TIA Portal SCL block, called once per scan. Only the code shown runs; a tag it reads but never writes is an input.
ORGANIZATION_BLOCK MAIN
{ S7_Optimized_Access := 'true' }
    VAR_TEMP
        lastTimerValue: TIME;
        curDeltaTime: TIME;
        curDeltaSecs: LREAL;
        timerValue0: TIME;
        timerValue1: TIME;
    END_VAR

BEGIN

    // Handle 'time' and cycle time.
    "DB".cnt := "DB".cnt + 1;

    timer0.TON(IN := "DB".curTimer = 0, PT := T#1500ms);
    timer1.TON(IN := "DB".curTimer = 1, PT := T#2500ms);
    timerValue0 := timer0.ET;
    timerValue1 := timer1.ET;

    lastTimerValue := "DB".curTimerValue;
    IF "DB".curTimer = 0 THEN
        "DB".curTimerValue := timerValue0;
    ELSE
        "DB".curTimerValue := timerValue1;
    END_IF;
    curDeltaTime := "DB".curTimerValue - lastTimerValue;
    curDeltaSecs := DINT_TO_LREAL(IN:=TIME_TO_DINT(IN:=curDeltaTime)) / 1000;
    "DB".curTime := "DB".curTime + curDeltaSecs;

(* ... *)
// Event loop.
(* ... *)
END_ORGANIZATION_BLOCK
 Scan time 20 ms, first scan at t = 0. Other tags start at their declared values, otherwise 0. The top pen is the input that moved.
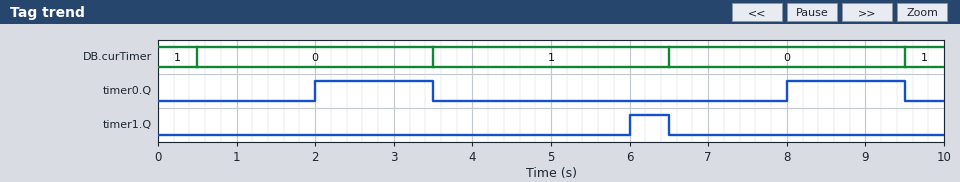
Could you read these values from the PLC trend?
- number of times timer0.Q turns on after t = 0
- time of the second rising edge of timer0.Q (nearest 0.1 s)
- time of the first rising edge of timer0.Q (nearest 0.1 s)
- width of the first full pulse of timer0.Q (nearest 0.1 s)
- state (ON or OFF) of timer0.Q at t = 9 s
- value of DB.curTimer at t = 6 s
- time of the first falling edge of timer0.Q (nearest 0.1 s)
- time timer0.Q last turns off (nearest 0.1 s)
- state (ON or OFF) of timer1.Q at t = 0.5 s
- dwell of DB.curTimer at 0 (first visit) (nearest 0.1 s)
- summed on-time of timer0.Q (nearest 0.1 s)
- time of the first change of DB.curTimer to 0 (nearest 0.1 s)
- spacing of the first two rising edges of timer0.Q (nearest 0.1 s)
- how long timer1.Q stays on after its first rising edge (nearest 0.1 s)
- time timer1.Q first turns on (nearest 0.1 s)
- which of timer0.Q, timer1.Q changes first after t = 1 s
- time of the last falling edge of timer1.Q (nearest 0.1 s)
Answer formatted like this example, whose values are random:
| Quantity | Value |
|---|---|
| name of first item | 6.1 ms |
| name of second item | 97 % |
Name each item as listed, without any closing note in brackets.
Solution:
| Quantity | Value |
|---|---|
| number of times timer0.Q turns on after t = 0 | 2 |
| time of the second rising edge of timer0.Q | 8.0 s |
| time of the first rising edge of timer0.Q | 2.0 s |
| width of the first full pulse of timer0.Q | 1.5 s |
| state (ON or OFF) of timer0.Q at t = 9 s | ON |
| value of DB.curTimer at t = 6 s | 1 |
| time of the first falling edge of timer0.Q | 3.5 s |
| time timer0.Q last turns off | 9.5 s |
| state (ON or OFF) of timer1.Q at t = 0.5 s | OFF |
| dwell of DB.curTimer at 0 (first visit) | 3.0 s |
| summed on-time of timer0.Q | 3.0 s |
| time of the first change of DB.curTimer to 0 | 0.5 s |
| spacing of the first two rising edges of timer0.Q | 6.0 s |
| how long timer1.Q stays on after its first rising edge | 0.5 s |
| time timer1.Q first turns on | 6.0 s |
| which of timer0.Q, timer1.Q changes first after t = 1 s | timer0.Q |
| time of the last falling edge of timer1.Q | 6.5 s |
